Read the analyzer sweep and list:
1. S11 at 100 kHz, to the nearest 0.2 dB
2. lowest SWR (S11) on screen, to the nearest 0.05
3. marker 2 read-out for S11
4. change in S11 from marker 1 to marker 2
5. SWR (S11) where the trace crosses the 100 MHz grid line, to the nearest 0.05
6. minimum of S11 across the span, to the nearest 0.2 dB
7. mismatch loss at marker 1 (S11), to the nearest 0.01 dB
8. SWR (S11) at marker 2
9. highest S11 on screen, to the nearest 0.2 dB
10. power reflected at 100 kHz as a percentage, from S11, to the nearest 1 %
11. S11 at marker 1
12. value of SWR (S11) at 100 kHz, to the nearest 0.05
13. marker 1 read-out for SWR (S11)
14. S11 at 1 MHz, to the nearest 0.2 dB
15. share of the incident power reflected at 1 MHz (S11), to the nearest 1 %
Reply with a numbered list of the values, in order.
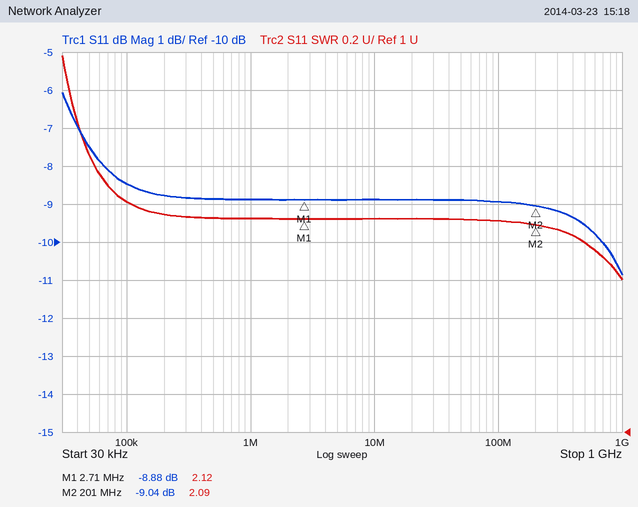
1. -8.4 dB
2. 1.80
3. -9.04 dB
4. -0.16 dB
5. 2.10
6. -10.8 dB
7. 0.60 dB
8. 2.09
9. -6.0 dB
10. 14 %
11. -8.88 dB
12. 2.20
13. 2.12
14. -8.8 dB
15. 13 %
